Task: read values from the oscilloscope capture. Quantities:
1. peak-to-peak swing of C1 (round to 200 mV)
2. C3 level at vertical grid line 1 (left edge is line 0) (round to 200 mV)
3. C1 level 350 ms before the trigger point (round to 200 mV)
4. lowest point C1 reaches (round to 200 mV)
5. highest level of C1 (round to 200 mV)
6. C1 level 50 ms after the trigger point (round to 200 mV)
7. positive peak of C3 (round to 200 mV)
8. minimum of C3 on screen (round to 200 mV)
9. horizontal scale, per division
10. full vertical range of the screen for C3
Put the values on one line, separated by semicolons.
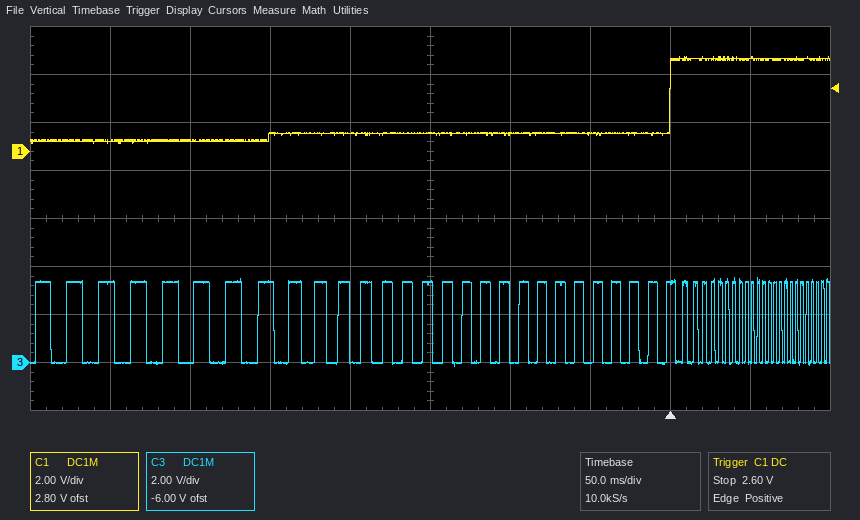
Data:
3.6 V; 3.4 V; 400 mV; 400 mV; 4.0 V; 3.8 V; 3.6 V; -200 mV; 50 ms; 16 V
